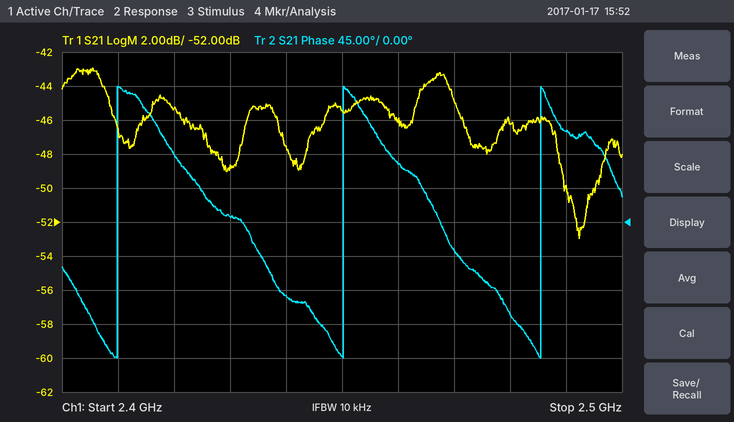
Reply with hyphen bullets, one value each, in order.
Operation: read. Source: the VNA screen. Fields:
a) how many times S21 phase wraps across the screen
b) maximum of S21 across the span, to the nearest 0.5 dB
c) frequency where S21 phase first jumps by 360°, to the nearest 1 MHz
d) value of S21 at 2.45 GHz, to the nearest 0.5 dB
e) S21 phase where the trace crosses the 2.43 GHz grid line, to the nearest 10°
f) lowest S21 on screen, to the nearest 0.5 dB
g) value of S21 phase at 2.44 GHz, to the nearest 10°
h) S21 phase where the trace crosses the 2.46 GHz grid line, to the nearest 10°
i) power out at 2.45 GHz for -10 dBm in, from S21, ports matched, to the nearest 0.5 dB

- 3
- -43.0 dB
- 2.410 GHz
- -45.5 dB
- 10°
- -53.0 dB
- -100°
- 80°
- -55.5 dBm
